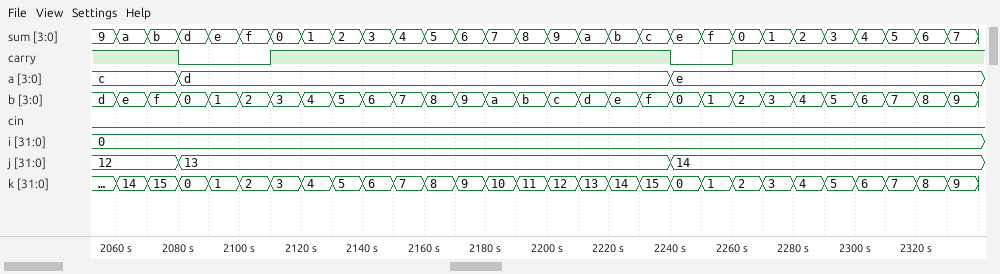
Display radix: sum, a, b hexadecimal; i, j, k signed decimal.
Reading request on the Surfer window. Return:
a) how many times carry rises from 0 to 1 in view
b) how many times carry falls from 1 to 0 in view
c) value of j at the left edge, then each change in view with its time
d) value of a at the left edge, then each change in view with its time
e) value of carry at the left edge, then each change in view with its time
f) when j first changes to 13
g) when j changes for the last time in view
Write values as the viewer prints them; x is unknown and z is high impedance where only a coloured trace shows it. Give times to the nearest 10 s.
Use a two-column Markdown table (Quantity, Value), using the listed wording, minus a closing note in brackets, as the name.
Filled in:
| Quantity | Value |
|---|---|
| how many times carry rises from 0 to 1 in view | 2 |
| how many times carry falls from 1 to 0 in view | 2 |
| value of j at the left edge, then each change in view with its time | 12, 13 at 2080 s, 14 at 2240 s |
| value of a at the left edge, then each change in view with its time | c, d at 2080 s, e at 2240 s |
| value of carry at the left edge, then each change in view with its time | 1, 0 at 2080 s, 1 at 2110 s, 0 at 2240 s, 1 at 2260 s |
| when j first changes to 13 | 2080 s |
| when j changes for the last time in view | 2240 s |
